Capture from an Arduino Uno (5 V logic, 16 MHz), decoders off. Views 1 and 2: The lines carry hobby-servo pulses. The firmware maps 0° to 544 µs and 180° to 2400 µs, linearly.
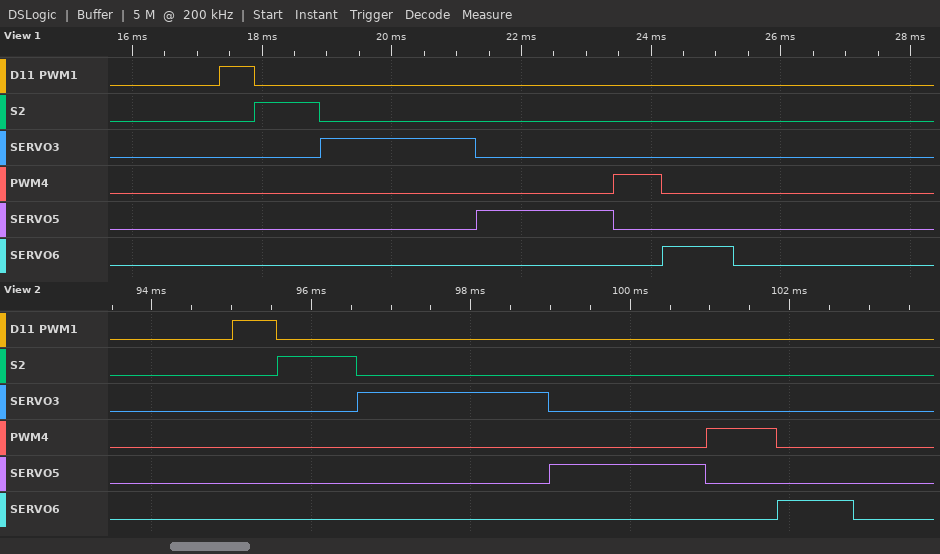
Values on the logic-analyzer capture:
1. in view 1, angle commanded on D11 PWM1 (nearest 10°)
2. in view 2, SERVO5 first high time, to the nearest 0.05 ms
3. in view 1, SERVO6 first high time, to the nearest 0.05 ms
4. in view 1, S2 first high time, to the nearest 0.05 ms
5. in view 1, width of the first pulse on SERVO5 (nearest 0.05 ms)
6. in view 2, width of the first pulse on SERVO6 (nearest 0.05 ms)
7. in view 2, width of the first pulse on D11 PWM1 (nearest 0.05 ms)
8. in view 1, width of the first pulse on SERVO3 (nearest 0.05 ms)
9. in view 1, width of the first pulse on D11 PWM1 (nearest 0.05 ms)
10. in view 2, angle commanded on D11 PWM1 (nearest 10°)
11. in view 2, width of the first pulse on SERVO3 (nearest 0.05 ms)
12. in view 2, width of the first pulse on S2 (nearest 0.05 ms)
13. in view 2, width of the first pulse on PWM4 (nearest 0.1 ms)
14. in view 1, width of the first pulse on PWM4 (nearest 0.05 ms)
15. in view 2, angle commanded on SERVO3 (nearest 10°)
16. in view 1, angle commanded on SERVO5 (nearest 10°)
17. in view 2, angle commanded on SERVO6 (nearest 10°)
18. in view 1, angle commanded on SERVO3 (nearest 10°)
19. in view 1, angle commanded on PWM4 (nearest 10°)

0°
1.95 ms
1.10 ms
1.00 ms
2.10 ms
0.95 ms
0.55 ms
2.40 ms
0.55 ms
0°
2.40 ms
1.00 ms
0.9 ms
0.75 ms
180°
150°
40°
180°
20°
